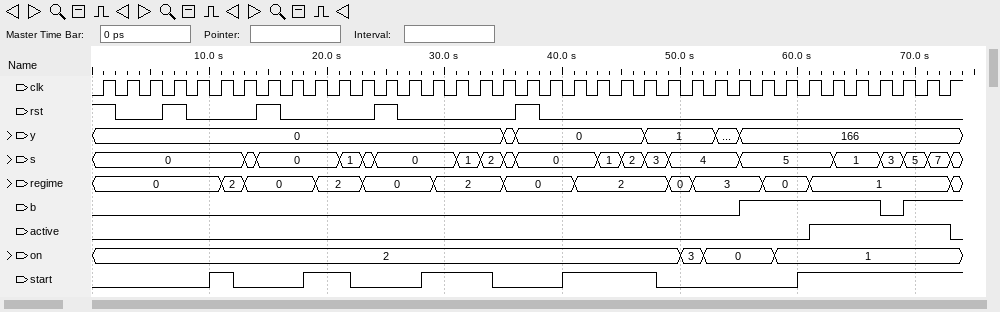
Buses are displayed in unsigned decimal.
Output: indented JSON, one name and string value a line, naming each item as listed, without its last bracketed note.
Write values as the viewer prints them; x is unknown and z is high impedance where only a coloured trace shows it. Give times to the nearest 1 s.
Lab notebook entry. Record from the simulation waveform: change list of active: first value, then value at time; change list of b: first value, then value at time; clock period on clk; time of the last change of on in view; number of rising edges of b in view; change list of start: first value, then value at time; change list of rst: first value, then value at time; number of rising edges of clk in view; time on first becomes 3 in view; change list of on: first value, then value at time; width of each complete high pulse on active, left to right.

{
  "change list of active: first value, then value at time": "0, 1 at 61 s, 0 at 73 s",
  "change list of b: first value, then value at time": "0, 1 at 55 s, 0 at 67 s, 1 at 69 s",
  "clock period on clk": "2 s",
  "time of the last change of on in view": "58 s",
  "number of rising edges of b in view": "2",
  "change list of start: first value, then value at time": "0, 1 at 10 s, 0 at 12 s, 1 at 18 s, 0 at 22 s, 1 at 28 s, 0 at 34 s, 1 at 40 s, 0 at 48 s, 1 at 60 s",
  "change list of rst: first value, then value at time": "1, 0 at 2 s, 1 at 6 s, 0 at 8 s, 1 at 14 s, 0 at 16 s, 1 at 24 s, 0 at 26 s, 1 at 36 s, 0 at 38 s",
  "number of rising edges of clk in view": "37",
  "time on first becomes 3 in view": "50 s",
  "change list of on: first value, then value at time": "2, 3 at 50 s, 0 at 52 s, 1 at 58 s",
  "width of each complete high pulse on active, left to right": "12 s"
}
